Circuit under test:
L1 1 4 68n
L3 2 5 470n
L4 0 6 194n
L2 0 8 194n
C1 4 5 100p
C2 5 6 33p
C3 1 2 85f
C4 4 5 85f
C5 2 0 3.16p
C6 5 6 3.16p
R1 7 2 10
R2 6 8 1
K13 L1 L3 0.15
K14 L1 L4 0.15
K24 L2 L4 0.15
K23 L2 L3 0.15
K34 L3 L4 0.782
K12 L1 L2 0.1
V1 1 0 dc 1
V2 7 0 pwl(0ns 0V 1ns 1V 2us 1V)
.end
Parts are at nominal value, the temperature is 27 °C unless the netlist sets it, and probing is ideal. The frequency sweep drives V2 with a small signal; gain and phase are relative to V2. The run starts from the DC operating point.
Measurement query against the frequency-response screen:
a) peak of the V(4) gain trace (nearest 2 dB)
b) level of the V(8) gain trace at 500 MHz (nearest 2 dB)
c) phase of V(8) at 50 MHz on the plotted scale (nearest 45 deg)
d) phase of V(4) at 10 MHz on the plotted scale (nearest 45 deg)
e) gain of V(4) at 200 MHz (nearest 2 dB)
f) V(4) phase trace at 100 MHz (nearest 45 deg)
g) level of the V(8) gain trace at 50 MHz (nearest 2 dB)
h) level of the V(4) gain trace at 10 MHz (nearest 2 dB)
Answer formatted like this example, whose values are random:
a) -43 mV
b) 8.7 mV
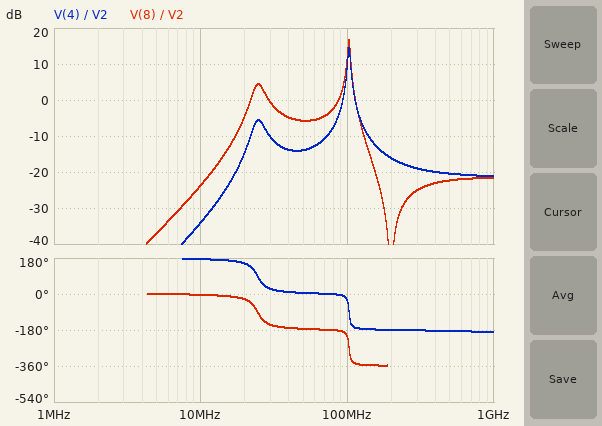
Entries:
a) 14 dB
b) -22 dB
c) -180 deg
d) 180 deg
e) -16 dB
f) -45 deg
g) -6 dB
h) -34 dB
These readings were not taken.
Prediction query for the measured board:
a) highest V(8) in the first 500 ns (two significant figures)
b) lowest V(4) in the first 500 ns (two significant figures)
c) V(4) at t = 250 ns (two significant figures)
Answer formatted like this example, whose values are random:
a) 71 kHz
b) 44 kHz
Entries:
a) 440 mV
b) 770 mV
c) 1.0 V
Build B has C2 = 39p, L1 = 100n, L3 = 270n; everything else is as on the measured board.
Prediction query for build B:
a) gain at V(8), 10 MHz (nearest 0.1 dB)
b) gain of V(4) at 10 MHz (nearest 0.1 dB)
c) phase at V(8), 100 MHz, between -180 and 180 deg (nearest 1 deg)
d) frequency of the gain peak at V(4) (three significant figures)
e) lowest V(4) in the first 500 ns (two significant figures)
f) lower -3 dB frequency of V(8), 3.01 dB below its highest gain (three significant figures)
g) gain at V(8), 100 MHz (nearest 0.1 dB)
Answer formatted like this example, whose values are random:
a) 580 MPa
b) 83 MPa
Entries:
a) -28.2 dB
b) -29.3 dB
c) 45 deg
d) 95.0 MHz
e) 640 mV
f) 90.9 MHz
g) 8.1 dB
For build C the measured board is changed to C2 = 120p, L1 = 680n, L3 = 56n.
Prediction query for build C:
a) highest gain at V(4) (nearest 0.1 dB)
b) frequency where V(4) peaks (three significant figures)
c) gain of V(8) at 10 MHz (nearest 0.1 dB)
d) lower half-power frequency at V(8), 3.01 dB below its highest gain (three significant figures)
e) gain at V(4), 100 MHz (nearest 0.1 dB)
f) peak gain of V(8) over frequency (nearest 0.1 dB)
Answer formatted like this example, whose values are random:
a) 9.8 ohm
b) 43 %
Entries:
a) 18.0 dB
b) 19.7 MHz
c) -30.6 dB
d) 51.5 MHz
e) 0.6 dB
f) 7.8 dB
